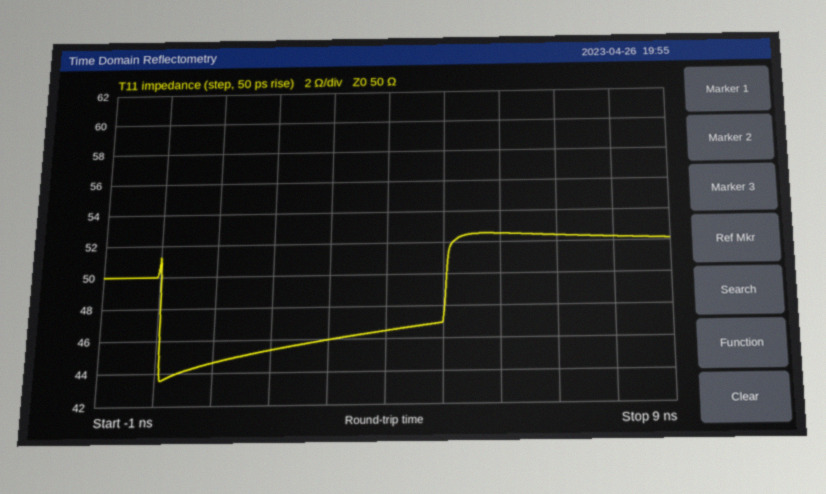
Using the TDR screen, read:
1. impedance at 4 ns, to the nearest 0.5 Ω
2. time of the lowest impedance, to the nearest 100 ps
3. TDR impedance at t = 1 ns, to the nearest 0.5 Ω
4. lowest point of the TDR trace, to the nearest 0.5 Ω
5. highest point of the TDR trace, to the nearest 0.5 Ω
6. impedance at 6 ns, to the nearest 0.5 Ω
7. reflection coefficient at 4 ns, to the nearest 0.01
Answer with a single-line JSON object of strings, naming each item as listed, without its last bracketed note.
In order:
{"impedance at 4 ns, to the nearest 0.5 Ω": "46.5 Ω", "time of the lowest impedance, to the nearest 100 ps": "100 ps", "TDR impedance at t = 1 ns, to the nearest 0.5 Ω": "44.5 Ω", "lowest point of the TDR trace, to the nearest 0.5 Ω": "43.5 Ω", "highest point of the TDR trace, to the nearest 0.5 Ω": "52.5 Ω", "impedance at 6 ns, to the nearest 0.5 Ω": "52.5 Ω", "reflection coefficient at 4 ns, to the nearest 0.01": "-0.04"}
